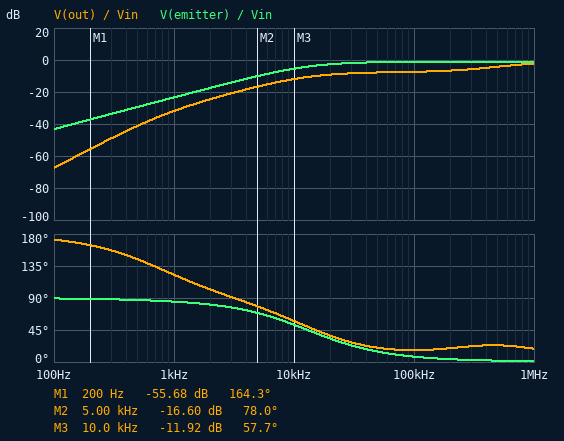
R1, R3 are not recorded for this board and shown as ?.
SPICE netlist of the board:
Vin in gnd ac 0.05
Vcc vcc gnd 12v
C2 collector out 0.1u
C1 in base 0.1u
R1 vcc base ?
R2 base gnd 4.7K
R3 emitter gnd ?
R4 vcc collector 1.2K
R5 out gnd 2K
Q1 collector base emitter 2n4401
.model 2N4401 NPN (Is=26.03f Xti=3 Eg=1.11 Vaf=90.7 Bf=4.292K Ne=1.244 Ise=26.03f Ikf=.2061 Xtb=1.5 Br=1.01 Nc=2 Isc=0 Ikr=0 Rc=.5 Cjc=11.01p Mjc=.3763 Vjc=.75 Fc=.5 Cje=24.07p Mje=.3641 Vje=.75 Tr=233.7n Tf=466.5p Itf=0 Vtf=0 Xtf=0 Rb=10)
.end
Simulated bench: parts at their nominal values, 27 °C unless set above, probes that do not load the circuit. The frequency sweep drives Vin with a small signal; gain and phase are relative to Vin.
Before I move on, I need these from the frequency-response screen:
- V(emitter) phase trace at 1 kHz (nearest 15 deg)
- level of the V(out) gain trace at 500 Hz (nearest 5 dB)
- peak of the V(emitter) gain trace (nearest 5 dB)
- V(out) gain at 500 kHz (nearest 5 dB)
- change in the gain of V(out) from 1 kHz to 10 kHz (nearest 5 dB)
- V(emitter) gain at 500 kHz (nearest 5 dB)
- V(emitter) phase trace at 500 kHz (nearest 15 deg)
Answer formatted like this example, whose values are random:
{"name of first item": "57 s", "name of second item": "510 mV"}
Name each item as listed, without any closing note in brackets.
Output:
{"V(emitter) phase trace at 1 kHz": "90 deg", "level of the V(out) gain trace at 500 Hz": "-40 dB", "peak of the V(emitter) gain trace": "0 dB", "V(out) gain at 500 kHz": "-5 dB", "change in the gain of V(out) from 1 kHz to 10 kHz": "20 dB", "V(emitter) gain at 500 kHz": "0 dB", "V(emitter) phase trace at 500 kHz": "0 deg"}
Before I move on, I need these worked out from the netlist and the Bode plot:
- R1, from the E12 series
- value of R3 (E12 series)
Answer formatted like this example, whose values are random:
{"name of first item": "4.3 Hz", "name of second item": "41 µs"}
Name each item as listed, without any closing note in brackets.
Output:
{"R1, from the E12 series": "12 kΩ", "value of R3": "120 Ω"}
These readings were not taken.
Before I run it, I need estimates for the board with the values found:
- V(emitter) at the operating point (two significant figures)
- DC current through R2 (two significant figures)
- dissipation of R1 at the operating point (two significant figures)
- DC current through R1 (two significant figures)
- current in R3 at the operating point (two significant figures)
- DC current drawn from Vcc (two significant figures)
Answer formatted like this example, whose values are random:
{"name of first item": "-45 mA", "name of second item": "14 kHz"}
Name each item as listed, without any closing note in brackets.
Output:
{"V(emitter) at the operating point": "1.1 V", "DC current through R2": "390 µA", "dissipation of R1 at the operating point": "8.6 mW", "DC current through R1": "850 µA", "current in R3 at the operating point": "9.4 mA", "DC current drawn from Vcc": "9.8 mA"}
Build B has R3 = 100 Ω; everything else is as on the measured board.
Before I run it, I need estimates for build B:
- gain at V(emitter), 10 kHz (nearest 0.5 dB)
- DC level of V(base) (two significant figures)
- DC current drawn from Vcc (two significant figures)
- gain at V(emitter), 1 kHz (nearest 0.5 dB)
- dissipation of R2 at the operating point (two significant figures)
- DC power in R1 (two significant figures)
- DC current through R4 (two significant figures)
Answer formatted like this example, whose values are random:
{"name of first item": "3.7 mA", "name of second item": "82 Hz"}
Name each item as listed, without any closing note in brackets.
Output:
{"gain at V(emitter), 10 kHz": "-6.5 dB", "DC level of V(base)": "1.7 V", "DC current drawn from Vcc": "10 mA", "gain at V(emitter), 1 kHz": "-25.0 dB", "dissipation of R2 at the operating point": "590 µW", "DC power in R1": "8.9 mW", "DC current through R4": "9.1 mA"}
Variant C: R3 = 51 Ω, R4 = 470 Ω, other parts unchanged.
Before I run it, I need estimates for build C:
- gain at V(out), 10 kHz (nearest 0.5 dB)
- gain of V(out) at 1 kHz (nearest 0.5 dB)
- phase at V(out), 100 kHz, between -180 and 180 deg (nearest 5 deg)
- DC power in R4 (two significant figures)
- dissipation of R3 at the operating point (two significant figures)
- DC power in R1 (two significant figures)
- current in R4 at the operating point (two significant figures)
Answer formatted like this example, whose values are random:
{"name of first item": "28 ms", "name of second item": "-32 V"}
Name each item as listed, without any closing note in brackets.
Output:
{"gain at V(out), 10 kHz": "-17.0 dB", "gain of V(out) at 1 kHz": "-38.5 dB", "phase at V(out), 100 kHz, between -180 and 180 deg": "170 deg", "DC power in R4": "240 mW", "dissipation of R3 at the operating point": "27 mW", "DC power in R1": "8.5 mW", "current in R4 at the operating point": "23 mA"}
